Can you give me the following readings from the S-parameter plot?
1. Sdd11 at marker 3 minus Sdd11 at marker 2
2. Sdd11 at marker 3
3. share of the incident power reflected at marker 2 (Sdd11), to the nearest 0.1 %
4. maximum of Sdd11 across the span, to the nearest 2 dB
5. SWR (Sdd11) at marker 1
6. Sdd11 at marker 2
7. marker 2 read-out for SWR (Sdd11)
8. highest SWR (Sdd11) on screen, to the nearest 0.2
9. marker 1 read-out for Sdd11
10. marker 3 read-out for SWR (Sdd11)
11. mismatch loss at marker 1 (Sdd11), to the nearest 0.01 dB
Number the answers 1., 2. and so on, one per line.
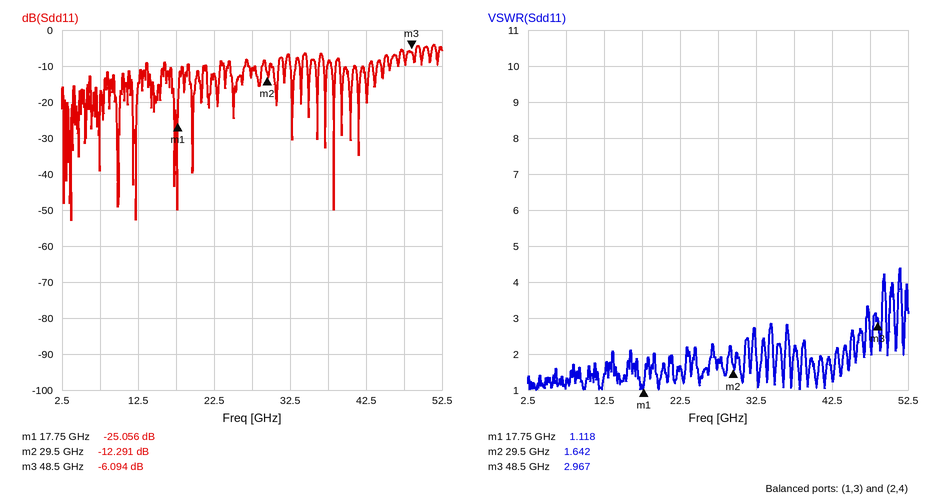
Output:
1. 6.197 dB
2. -6.094 dB
3. 5.9 %
4. -4 dB
5. 1.118
6. -12.291 dB
7. 1.642
8. 4.4
9. -25.056 dB
10. 2.967
11. 0.01 dB
